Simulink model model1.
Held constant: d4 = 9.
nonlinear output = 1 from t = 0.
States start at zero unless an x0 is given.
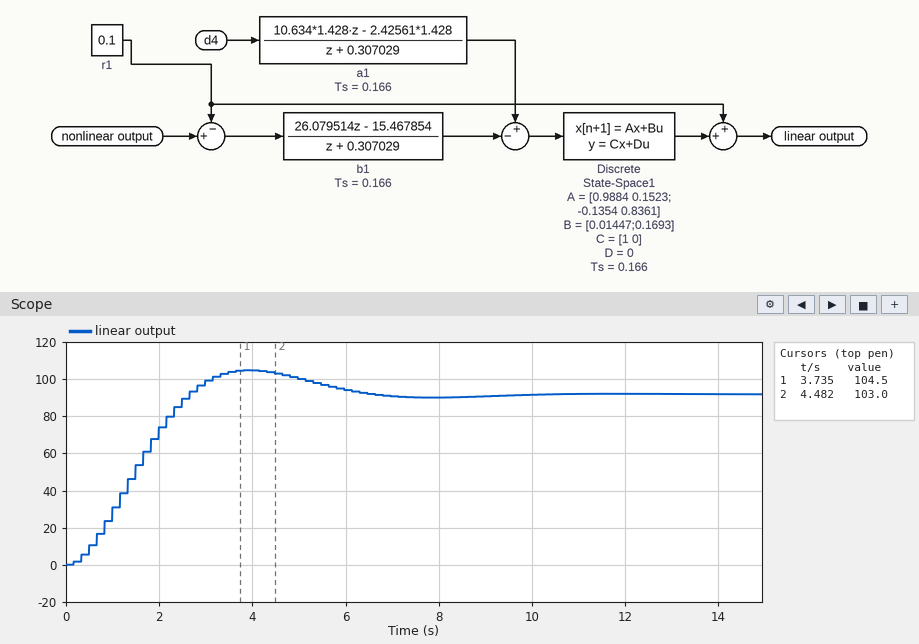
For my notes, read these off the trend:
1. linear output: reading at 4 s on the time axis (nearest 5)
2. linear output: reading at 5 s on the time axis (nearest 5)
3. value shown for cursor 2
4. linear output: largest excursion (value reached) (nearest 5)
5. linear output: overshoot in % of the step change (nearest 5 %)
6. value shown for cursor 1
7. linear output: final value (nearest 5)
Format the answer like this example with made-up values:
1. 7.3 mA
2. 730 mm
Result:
1. 105
2. 100
3. 103.0
4. 105
5. 15 %
6. 104.5
7. 90
